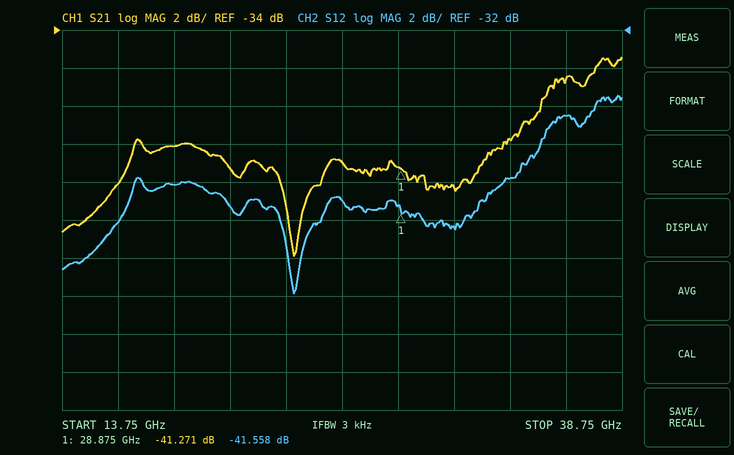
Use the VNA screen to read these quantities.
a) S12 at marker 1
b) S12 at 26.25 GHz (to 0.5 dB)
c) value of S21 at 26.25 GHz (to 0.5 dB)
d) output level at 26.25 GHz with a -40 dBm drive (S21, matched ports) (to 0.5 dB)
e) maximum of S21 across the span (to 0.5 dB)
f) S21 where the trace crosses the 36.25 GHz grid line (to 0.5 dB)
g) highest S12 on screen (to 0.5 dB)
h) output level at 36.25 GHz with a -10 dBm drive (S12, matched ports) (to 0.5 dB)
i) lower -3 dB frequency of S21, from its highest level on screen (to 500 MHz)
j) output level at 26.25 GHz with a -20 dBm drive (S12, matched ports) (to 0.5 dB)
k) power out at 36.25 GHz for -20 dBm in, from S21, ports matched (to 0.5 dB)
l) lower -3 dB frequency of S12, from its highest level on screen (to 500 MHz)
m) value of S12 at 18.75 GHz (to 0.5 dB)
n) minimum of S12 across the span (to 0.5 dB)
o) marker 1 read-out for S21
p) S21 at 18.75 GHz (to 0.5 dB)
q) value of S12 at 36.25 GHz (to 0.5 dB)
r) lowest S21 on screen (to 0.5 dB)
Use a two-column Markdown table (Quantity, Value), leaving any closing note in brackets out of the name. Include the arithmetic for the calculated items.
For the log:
| Quantity | Value |
|---|---|
| S12 at marker 1 | -41.558 dB |
| S12 at 26.25 GHz | -41.0 dB |
| value of S21 at 26.25 GHz | -41.0 dB |
| output level at 26.25 GHz with a -40 dBm drive (S21, matched ports) | -40 dBm + (-41.0 dB) = -81.0 dBm |
| maximum of S21 across the span | -35.5 dB |
| S21 where the trace crosses the 36.25 GHz grid line | -36.5 dB |
| highest S12 on screen | -35.5 dB |
| output level at 36.25 GHz with a -10 dBm drive (S12, matched ports) | -10 dBm + (-36.5 dB) = -46.5 dBm |
| lower -3 dB frequency of S21, from its highest level on screen | 35.0 GHz |
| output level at 26.25 GHz with a -20 dBm drive (S12, matched ports) | -20 dBm + (-41.0 dB) = -61.0 dBm |
| power out at 36.25 GHz for -20 dBm in, from S21, ports matched | -20 dBm + (-36.5 dB) = -56.5 dBm |
| lower -3 dB frequency of S12, from its highest level on screen | 35.0 GHz |
| value of S12 at 18.75 GHz | -40.0 dB |
| minimum of S12 across the span | -46.0 dB |
| marker 1 read-out for S21 | -41.271 dB |
| S21 at 18.75 GHz | -40.0 dB |
| value of S12 at 36.25 GHz | -36.5 dB |
| lowest S21 on screen | -46.0 dB |
